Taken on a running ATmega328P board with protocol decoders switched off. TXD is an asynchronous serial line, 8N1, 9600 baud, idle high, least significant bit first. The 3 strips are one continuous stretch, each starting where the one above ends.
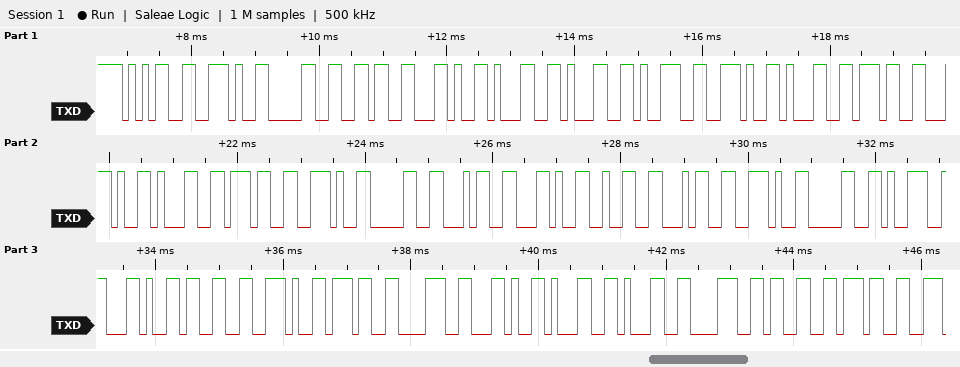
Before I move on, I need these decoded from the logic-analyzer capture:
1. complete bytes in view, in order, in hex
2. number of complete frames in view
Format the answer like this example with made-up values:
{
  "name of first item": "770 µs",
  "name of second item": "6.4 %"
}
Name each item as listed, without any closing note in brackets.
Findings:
{
  "complete bytes in view, in order, in hex": "35 2E 30 36 2C 31 31 39 2E 31 37 2C 31 37 2E 30 34 2C 32 34 2E 30 39 2C 33 2E 37 38 2C 31 31 38 33 37",
  "number of complete frames in view": "34"
}
